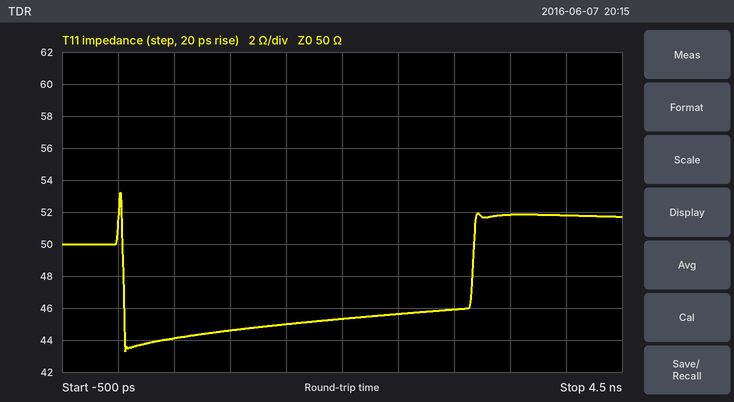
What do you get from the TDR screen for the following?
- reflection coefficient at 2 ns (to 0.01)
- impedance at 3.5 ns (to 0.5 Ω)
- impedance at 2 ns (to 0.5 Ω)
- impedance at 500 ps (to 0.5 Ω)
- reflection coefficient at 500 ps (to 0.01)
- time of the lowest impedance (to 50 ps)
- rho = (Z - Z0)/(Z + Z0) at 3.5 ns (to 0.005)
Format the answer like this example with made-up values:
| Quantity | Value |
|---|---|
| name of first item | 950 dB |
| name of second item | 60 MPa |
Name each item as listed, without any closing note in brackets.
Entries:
| Quantity | Value |
|---|---|
| reflection coefficient at 2 ns | -0.05 |
| impedance at 3.5 ns | 52.0 Ω |
| impedance at 2 ns | 45.5 Ω |
| impedance at 500 ps | 44.0 Ω |
| reflection coefficient at 500 ps | -0.06 |
| time of the lowest impedance | 50 ps |
| rho = (Z - Z0)/(Z + Z0) at 3.5 ns | +0.020 |
